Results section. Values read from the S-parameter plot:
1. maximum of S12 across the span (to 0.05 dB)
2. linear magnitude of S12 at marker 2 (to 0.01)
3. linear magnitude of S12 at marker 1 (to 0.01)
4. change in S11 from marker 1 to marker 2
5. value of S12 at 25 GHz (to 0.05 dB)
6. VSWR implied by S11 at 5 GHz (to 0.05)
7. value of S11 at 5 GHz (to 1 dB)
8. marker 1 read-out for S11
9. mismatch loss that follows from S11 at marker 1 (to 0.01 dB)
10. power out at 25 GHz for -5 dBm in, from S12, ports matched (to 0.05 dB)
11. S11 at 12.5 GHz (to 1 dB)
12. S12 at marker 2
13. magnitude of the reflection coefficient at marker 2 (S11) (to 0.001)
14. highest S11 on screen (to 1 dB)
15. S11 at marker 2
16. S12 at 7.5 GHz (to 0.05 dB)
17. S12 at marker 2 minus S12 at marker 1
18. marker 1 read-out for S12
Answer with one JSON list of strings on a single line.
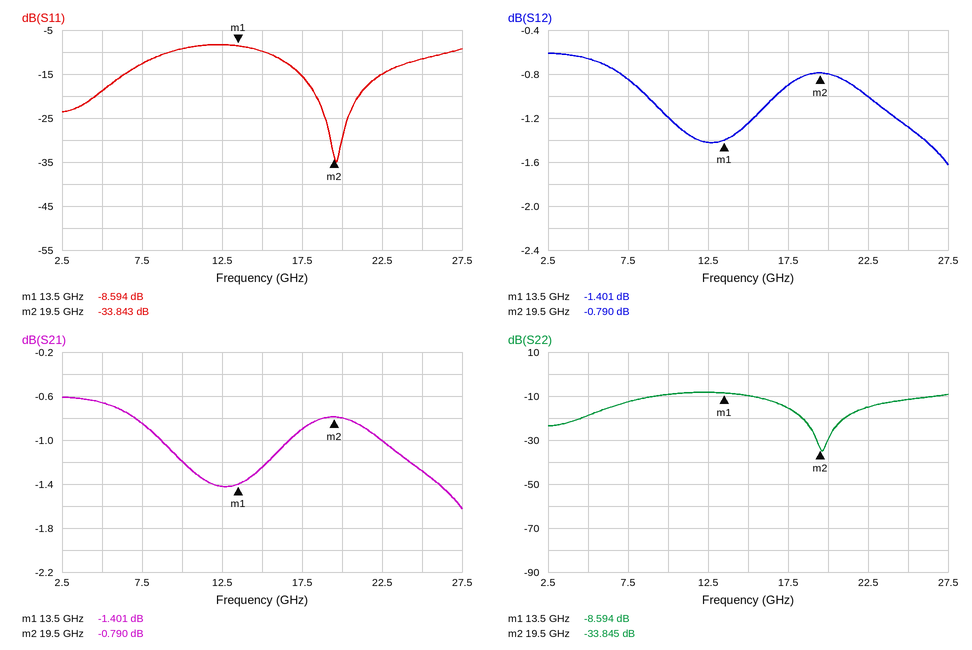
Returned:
["-0.60 dB", "0.91", "0.85", "-25.249 dB", "-1.30 dB", "1.25", "-19 dB", "-8.594 dB", "0.65 dB", "-6.30 dBm", "-8 dB", "-0.790 dB", "0.020", "-8 dB", "-33.843 dB", "-0.85 dB", "0.611 dB", "-1.401 dB"]
